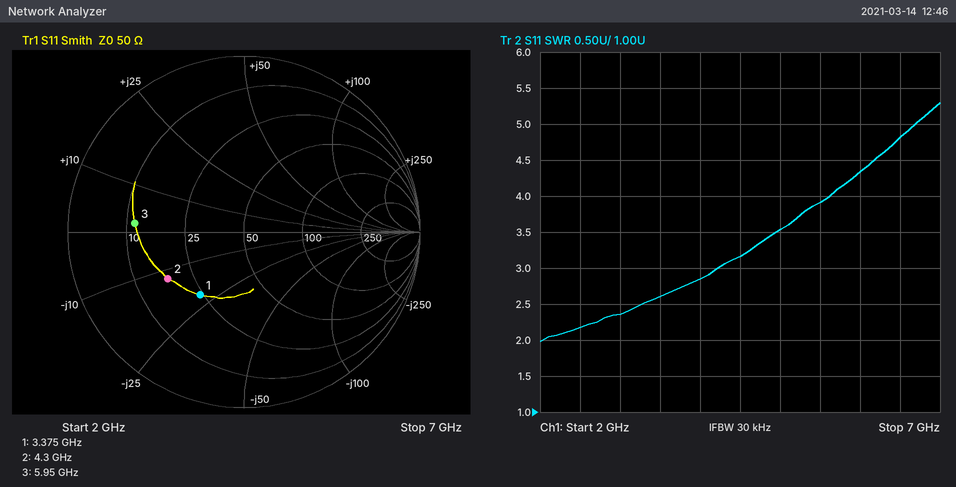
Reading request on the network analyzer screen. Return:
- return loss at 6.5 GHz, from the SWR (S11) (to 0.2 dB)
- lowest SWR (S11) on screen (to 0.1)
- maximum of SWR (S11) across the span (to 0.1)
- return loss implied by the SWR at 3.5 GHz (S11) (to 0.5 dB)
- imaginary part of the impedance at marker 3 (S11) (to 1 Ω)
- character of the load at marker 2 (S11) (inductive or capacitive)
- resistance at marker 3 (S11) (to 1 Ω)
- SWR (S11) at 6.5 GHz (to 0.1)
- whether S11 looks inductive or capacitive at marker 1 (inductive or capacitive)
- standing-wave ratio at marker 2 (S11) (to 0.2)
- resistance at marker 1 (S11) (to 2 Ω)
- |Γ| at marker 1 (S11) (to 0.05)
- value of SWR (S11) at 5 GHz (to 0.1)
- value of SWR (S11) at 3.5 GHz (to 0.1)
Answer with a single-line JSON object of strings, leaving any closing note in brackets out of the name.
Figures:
{"return loss at 6.5 GHz, from the SWR (S11)": "3.6 dB", "lowest SWR (S11) on screen": "2.0", "maximum of SWR (S11) across the span": "5.3", "return loss implied by the SWR at 3.5 GHz (S11)": "7.0 dB", "imaginary part of the impedance at marker 3 (S11)": "+2 Ω", "character of the load at marker 2 (S11)": "capacitive", "resistance at marker 3 (S11)": "12 Ω", "SWR (S11) at 6.5 GHz": "4.8", "whether S11 looks inductive or capacitive at marker 1": "capacitive", "standing-wave ratio at marker 2 (S11)": "3.0", "resistance at marker 1 (S11)": "24 Ω", "|Γ| at marker 1 (S11)": "0.45", "value of SWR (S11) at 5 GHz": "3.5", "value of SWR (S11) at 3.5 GHz": "2.6"}
